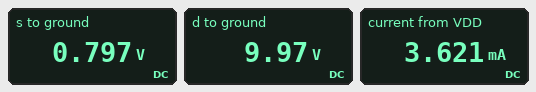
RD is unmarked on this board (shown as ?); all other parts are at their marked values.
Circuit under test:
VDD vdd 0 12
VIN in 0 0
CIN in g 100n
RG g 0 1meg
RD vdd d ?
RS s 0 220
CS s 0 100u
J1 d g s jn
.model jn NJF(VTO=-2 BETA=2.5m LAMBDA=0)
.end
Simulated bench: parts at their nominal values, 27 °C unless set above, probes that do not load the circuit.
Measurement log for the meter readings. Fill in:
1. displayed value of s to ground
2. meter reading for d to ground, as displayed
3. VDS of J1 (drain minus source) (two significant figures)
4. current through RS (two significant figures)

0.797 V
9.97 V
9.2 V
3.6 mA
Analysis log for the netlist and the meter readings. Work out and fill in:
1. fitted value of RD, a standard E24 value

560 Ω
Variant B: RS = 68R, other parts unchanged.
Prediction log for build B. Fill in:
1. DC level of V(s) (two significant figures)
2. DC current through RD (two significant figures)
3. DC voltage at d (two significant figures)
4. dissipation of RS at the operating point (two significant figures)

420 mV
6.2 mA
8.5 V
2.6 mW
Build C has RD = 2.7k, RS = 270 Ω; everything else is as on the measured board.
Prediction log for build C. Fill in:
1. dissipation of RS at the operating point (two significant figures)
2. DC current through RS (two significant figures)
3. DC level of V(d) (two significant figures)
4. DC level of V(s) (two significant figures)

2.8 mW
3.2 mA
3.3 V
870 mV
